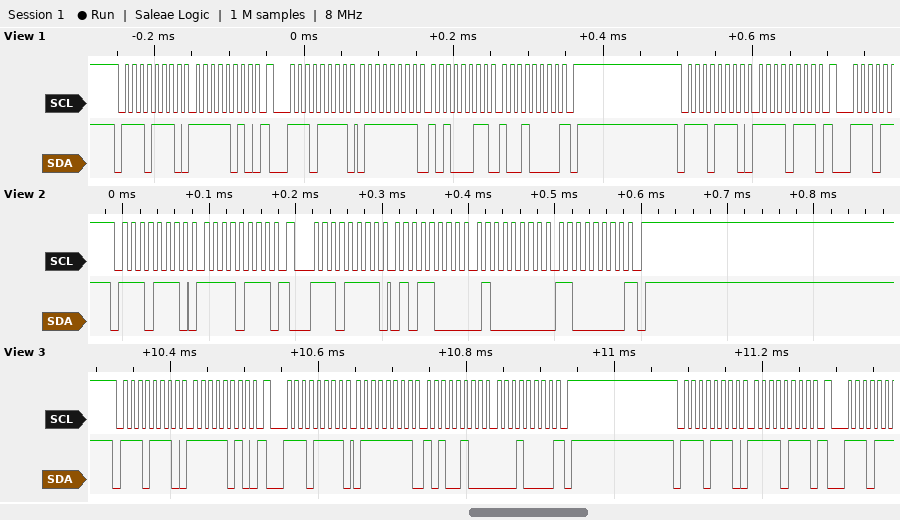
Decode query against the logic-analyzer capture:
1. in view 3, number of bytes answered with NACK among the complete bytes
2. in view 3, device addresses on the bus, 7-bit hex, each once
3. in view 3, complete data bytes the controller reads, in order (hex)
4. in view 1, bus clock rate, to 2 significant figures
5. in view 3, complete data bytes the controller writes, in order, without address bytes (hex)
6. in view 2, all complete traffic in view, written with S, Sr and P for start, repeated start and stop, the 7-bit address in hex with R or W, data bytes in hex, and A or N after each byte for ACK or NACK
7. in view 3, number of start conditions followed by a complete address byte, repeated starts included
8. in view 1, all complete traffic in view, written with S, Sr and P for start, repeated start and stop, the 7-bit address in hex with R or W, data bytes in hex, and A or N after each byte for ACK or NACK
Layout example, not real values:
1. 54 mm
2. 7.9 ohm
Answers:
1. 1
2. 0x77
3. 7F A4 10
4. 100 kHz
5. FA F7
6. S 77W A F7 A Sr 77R A 58 A 40 A C0 N P
7. 3
8. S 77W A FA A Sr 77R A 7F A A3 A 90 N P S 77W A F7 A
